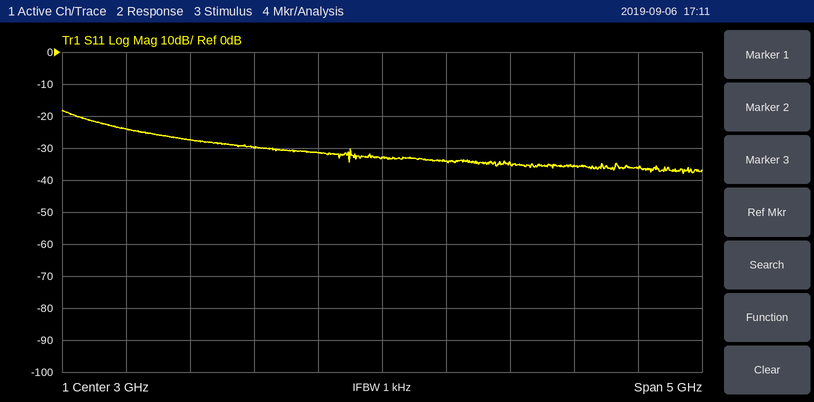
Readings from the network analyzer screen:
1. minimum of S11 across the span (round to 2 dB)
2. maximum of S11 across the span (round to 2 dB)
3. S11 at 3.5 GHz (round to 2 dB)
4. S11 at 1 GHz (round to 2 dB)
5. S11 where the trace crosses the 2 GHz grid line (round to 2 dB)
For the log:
-38 dB
-18 dB
-34 dB
-24 dB
-30 dB
